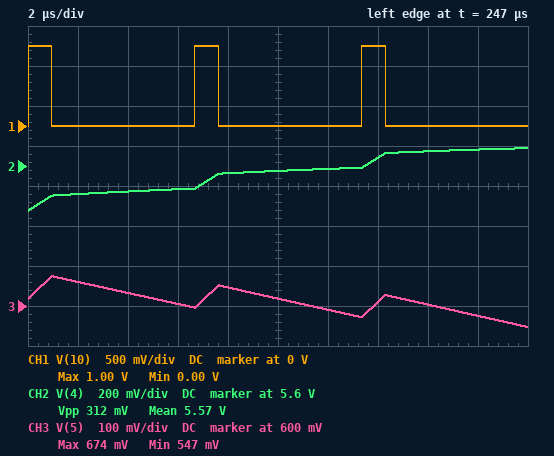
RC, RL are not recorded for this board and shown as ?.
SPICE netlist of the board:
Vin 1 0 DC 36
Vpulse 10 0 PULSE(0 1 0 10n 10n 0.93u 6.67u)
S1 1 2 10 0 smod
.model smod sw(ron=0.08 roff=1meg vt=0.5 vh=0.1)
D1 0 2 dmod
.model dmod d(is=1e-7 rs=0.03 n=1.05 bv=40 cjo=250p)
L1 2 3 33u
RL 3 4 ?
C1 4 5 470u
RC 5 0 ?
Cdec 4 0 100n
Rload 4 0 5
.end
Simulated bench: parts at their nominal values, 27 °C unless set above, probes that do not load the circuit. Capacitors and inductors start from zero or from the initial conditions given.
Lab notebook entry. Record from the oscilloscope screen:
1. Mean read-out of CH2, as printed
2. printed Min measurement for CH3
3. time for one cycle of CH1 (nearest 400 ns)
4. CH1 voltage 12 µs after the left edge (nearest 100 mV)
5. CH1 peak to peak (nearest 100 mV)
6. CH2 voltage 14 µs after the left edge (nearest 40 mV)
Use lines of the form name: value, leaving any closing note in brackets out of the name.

Mean read-out of CH2, as printed: 5.57 V
printed Min measurement for CH3: 547 mV
time for one cycle of CH1: 6.8 µs
CH1 voltage 12 µs after the left edge: 0 V
CH1 peak to peak: 1.0 V
CH2 voltage 14 µs after the left edge: 5.64 V
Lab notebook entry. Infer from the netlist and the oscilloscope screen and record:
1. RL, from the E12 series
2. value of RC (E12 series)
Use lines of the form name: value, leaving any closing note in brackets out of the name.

RL, from the E12 series: 0.033 Ω
value of RC: 0.068 Ω
